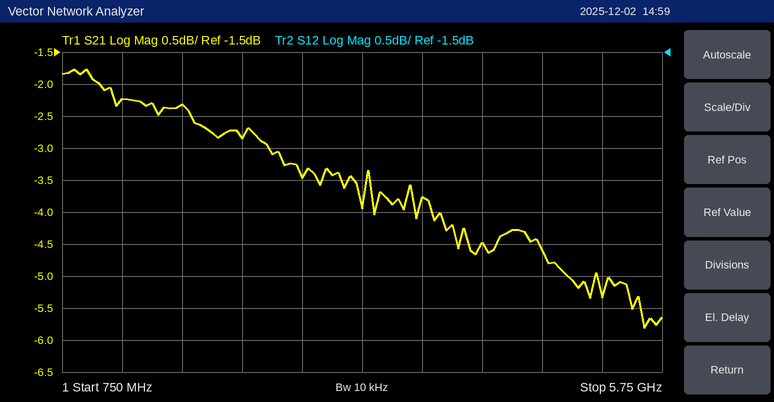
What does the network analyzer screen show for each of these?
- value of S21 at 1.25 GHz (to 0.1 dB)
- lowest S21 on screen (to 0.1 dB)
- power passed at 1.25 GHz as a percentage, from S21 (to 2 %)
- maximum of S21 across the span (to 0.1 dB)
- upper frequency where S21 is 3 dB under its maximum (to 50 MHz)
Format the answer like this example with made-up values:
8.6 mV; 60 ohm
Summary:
-2.2 dB; -5.8 dB; 60 %; -1.8 dB; 4.80 GHz
